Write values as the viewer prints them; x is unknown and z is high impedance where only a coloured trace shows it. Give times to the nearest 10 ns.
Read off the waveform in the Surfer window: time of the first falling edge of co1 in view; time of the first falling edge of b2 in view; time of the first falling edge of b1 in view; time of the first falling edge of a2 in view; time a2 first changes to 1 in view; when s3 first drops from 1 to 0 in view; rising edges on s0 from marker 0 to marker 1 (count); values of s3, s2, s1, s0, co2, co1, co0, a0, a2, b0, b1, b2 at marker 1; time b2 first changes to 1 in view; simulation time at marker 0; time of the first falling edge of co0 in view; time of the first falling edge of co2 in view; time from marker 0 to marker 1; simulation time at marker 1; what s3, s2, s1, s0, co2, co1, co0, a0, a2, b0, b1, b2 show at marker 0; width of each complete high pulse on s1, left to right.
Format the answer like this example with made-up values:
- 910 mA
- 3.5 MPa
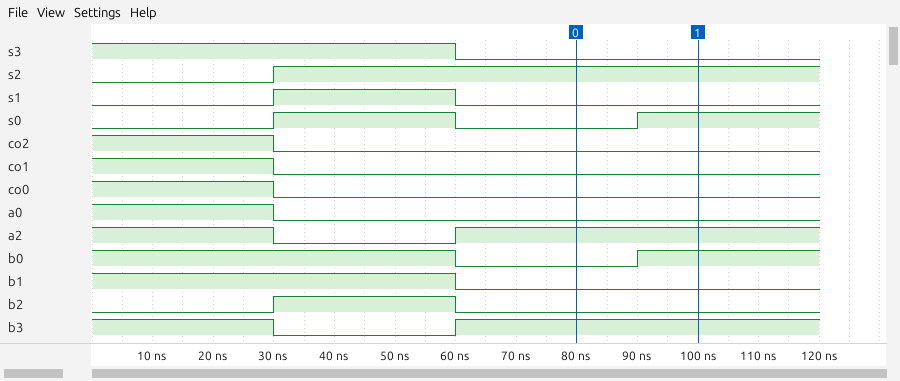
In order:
- 30 ns
- 60 ns
- 60 ns
- 30 ns
- 60 ns
- 60 ns
- 1
- s3=0, s2=1, s1=0, s0=1, co2=0, co1=0, co0=0, a0=0, a2=1, b0=1, b1=0, b2=0
- 30 ns
- 80 ns
- 30 ns
- 30 ns
- 20 ns
- 100 ns
- s3=0, s2=1, s1=0, s0=0, co2=0, co1=0, co0=0, a0=0, a2=1, b0=0, b1=0, b2=0
- 30 ns
